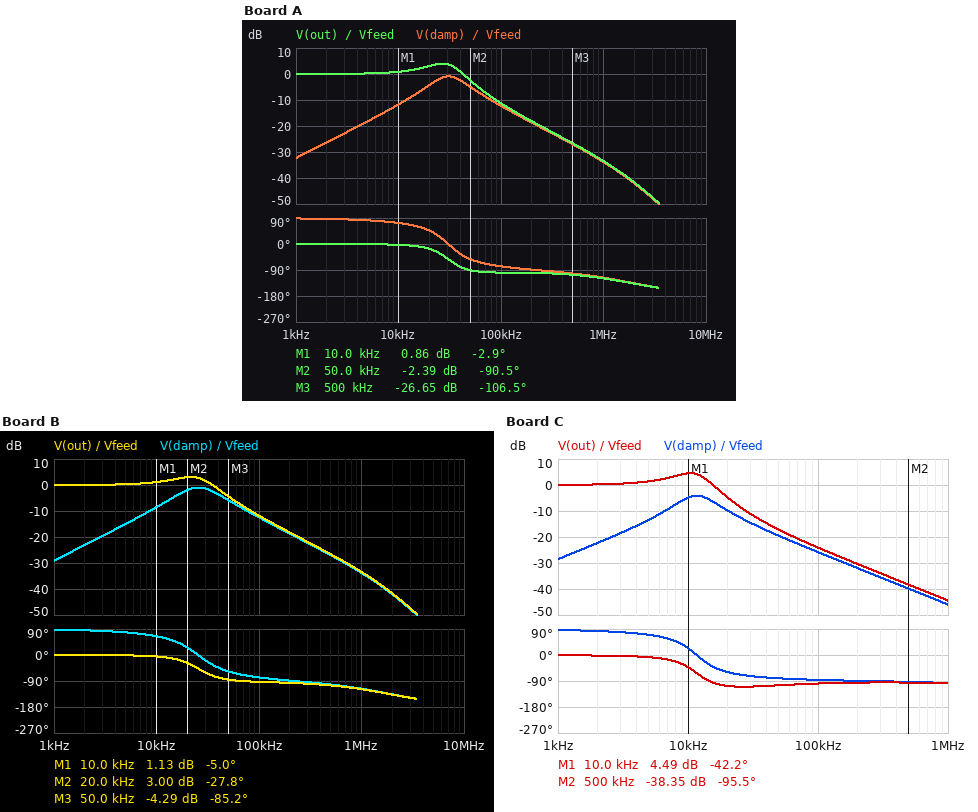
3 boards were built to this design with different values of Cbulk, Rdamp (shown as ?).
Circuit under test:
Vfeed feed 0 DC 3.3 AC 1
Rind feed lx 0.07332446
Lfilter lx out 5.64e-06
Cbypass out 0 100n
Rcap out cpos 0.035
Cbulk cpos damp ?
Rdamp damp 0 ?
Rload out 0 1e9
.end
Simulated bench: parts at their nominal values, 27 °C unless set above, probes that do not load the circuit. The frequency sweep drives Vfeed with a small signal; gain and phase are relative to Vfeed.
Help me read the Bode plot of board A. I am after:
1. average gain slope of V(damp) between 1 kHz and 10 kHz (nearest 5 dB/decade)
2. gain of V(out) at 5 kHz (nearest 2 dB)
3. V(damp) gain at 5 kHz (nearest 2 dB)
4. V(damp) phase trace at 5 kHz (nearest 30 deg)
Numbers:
20 dB/decade
0 dB
-18 dB
90 deg
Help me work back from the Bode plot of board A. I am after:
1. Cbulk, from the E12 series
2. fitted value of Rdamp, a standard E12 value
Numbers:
4.7 µF
0.82 Ω
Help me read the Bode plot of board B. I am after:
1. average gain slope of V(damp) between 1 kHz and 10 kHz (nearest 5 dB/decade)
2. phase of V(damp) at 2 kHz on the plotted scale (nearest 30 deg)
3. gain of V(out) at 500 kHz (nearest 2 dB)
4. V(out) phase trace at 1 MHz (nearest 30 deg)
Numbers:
20 dB/decade
90 deg
-26 dB
-120 deg
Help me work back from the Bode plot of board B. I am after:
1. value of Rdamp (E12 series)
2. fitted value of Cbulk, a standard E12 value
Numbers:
0.82 Ω
6.8 µF
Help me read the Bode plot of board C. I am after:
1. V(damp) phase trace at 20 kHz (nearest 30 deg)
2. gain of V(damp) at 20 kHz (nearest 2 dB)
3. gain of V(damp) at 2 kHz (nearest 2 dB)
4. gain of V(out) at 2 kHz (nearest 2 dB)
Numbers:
-60 deg
-10 dB
-22 dB
0 dB
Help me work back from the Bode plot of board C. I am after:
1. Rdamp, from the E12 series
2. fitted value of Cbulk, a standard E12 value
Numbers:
0.18 Ω
33 µF
